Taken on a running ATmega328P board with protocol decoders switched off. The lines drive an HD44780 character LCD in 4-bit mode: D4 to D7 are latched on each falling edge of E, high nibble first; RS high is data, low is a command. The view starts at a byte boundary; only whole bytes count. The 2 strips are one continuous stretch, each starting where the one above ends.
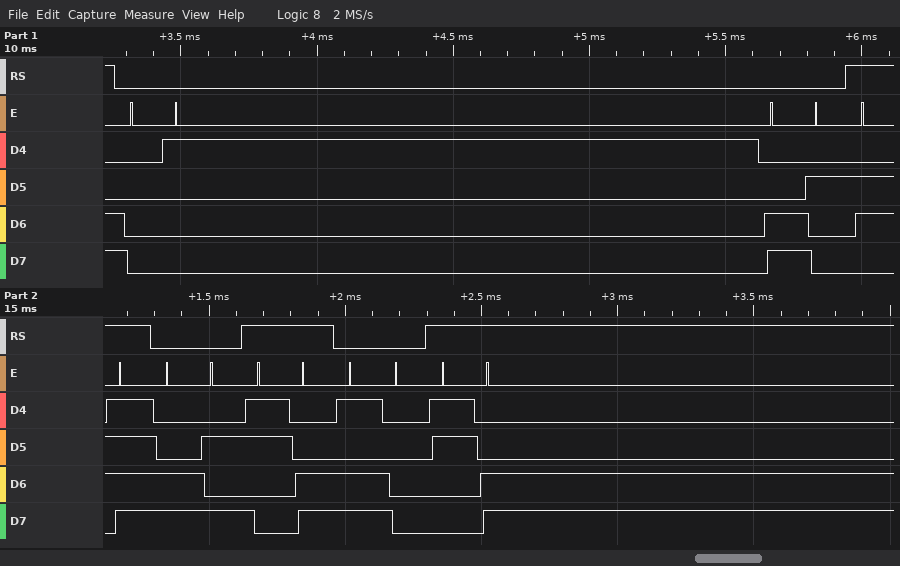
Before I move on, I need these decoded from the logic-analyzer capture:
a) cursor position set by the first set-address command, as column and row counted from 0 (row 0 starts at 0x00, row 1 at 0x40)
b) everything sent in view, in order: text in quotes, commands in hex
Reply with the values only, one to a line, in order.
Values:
column 2, row 1
0x01 0xC2 "o" 0xCA "<" 0xD0 "<"
